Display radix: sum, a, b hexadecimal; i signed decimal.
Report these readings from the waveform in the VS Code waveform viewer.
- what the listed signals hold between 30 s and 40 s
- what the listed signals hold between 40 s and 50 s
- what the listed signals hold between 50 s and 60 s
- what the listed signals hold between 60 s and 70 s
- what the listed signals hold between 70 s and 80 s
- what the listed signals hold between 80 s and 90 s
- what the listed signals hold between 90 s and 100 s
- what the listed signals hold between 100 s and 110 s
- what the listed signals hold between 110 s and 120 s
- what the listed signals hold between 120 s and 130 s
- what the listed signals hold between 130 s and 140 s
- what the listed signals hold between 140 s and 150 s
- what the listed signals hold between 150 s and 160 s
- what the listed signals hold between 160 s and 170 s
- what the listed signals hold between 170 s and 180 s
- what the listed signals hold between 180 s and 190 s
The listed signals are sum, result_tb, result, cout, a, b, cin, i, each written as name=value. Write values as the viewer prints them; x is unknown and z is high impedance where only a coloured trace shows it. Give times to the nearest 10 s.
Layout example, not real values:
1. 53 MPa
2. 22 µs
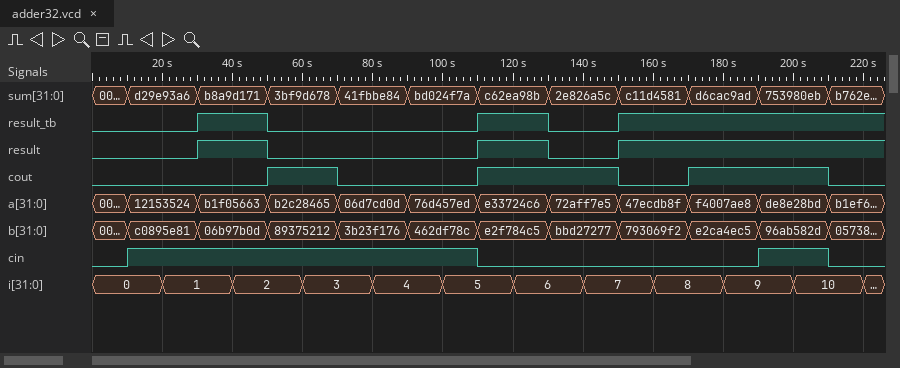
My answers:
1. sum=b8a9d171, result_tb=1, result=1, cout=0, a=b1f05663, b=06b97b0d, cin=1, i=1
2. sum=b8a9d171, result_tb=1, result=1, cout=0, a=b1f05663, b=06b97b0d, cin=1, i=2
3. sum=3bf9d678, result_tb=0, result=0, cout=1, a=b2c28465, b=89375212, cin=1, i=2
4. sum=3bf9d678, result_tb=0, result=0, cout=1, a=b2c28465, b=89375212, cin=1, i=3
5. sum=41fbbe84, result_tb=0, result=0, cout=0, a=06d7cd0d, b=3b23f176, cin=1, i=3
6. sum=41fbbe84, result_tb=0, result=0, cout=0, a=06d7cd0d, b=3b23f176, cin=1, i=4
7. sum=bd024f7a, result_tb=0, result=0, cout=0, a=76d457ed, b=462df78c, cin=1, i=4
8. sum=bd024f7a, result_tb=0, result=0, cout=0, a=76d457ed, b=462df78c, cin=1, i=5
9. sum=c62ea98b, result_tb=1, result=1, cout=1, a=e33724c6, b=e2f784c5, cin=0, i=5
10. sum=c62ea98b, result_tb=1, result=1, cout=1, a=e33724c6, b=e2f784c5, cin=0, i=6
11. sum=2e826a5c, result_tb=0, result=0, cout=1, a=72aff7e5, b=bbd27277, cin=0, i=6
12. sum=2e826a5c, result_tb=0, result=0, cout=1, a=72aff7e5, b=bbd27277, cin=0, i=7
13. sum=c11d4581, result_tb=1, result=1, cout=0, a=47ecdb8f, b=793069f2, cin=0, i=7
14. sum=c11d4581, result_tb=1, result=1, cout=0, a=47ecdb8f, b=793069f2, cin=0, i=8
15. sum=d6cac9ad, result_tb=1, result=1, cout=1, a=f4007ae8, b=e2ca4ec5, cin=0, i=8
16. sum=d6cac9ad, result_tb=1, result=1, cout=1, a=f4007ae8, b=e2ca4ec5, cin=0, i=9
